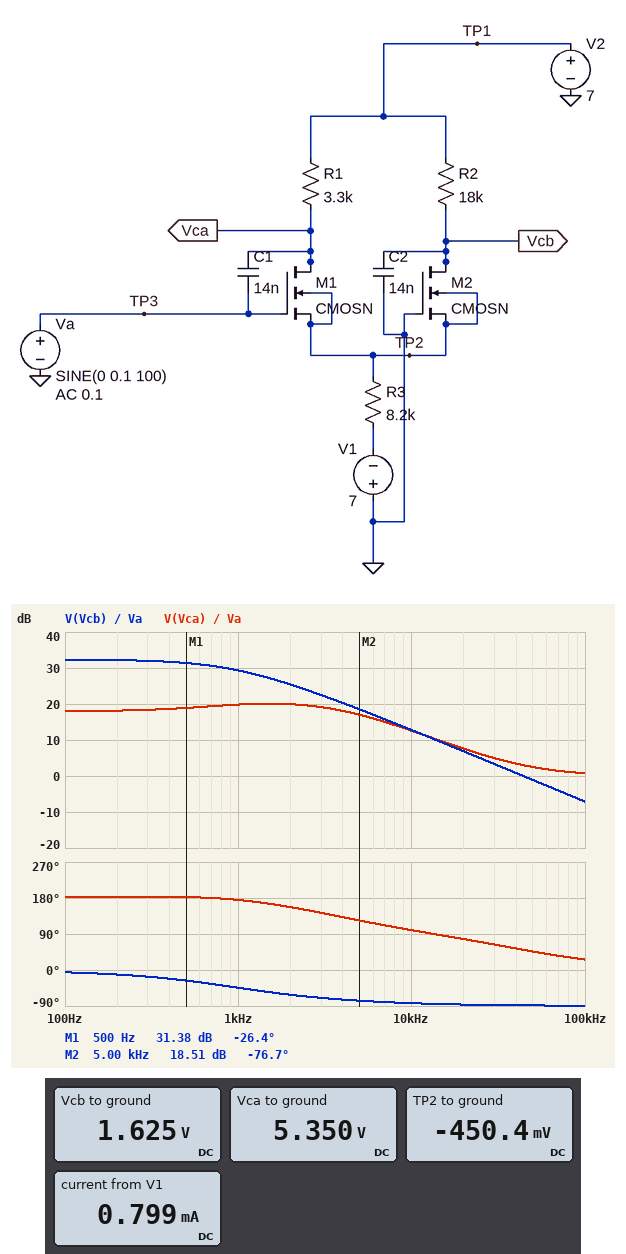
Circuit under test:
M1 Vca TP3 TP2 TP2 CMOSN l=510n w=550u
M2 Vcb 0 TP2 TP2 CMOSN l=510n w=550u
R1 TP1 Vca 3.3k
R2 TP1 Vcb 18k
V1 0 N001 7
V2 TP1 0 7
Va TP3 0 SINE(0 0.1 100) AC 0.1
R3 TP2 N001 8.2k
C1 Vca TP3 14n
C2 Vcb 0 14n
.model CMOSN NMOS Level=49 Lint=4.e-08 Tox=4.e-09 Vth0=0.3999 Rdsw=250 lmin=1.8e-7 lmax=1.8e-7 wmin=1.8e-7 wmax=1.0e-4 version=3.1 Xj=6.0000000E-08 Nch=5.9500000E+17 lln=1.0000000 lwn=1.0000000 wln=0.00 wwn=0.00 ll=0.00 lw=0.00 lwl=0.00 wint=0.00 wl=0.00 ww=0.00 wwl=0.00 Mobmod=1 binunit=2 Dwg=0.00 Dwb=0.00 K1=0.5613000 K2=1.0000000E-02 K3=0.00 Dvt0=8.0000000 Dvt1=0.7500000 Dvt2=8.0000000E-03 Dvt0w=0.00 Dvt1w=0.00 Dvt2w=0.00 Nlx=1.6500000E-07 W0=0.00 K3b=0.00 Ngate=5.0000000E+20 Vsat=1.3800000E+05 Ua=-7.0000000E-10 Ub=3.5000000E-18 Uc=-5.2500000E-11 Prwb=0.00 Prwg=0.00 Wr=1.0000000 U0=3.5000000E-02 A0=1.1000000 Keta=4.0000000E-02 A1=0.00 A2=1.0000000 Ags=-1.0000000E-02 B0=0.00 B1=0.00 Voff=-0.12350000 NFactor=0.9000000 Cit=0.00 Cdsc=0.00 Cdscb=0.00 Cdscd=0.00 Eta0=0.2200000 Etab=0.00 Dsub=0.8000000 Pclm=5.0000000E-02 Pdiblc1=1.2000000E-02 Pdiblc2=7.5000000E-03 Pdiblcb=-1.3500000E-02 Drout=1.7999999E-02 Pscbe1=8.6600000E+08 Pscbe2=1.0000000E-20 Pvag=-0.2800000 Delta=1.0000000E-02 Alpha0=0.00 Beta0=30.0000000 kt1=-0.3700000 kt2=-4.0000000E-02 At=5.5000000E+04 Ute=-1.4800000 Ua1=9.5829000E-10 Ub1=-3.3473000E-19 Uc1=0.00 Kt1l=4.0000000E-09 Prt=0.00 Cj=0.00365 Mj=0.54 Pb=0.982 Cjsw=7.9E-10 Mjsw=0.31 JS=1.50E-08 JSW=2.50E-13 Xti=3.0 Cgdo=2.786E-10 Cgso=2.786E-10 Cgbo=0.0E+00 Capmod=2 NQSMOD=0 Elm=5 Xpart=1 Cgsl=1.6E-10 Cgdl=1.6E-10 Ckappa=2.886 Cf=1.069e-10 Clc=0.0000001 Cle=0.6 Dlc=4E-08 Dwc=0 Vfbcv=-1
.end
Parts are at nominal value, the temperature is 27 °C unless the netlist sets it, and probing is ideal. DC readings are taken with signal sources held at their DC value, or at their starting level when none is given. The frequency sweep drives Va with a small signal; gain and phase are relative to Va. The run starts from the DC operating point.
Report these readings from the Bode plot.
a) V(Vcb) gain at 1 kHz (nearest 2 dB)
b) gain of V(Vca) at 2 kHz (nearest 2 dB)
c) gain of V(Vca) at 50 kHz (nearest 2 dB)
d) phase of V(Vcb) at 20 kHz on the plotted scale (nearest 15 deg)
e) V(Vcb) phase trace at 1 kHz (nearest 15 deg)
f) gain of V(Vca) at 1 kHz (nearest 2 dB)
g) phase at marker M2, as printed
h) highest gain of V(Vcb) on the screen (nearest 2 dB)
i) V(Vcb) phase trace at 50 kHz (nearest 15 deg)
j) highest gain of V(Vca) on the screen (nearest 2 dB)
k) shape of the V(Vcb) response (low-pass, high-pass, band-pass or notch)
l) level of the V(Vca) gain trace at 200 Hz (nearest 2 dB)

30 dB
20 dB
2 dB
-90 deg
-45 deg
20 dB
-76.7 deg
32 dB
-90 deg
20 dB
low-pass
18 dB
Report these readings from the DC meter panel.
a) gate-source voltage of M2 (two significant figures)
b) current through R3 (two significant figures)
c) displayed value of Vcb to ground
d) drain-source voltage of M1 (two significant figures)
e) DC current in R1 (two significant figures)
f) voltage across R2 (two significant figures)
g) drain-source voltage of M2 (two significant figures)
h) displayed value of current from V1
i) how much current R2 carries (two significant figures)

450 mV
800 µA
1.625 V
5.8 V
500 µA
5.4 V
2.1 V
0.799 mA
300 µA
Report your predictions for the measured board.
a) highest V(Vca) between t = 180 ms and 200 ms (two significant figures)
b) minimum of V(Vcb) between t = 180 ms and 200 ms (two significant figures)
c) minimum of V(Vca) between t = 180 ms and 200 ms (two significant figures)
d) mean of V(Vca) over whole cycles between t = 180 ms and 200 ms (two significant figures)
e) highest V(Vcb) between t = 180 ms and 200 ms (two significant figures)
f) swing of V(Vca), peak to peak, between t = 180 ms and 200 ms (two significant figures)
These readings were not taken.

5.8 V
-510 mV
4.6 V
5.3 V
5.4 V
1.2 V
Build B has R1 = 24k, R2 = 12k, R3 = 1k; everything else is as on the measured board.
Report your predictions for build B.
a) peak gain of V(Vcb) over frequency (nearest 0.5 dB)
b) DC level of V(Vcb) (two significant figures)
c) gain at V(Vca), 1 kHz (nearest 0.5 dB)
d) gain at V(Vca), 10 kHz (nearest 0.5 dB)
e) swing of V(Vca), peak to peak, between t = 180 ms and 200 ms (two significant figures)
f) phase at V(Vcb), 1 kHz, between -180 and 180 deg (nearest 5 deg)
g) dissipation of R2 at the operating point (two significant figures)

-6.0 dB
-5.4 V
-22.0 dB
-7.5 dB
1.6 mV
80 deg
13 mW
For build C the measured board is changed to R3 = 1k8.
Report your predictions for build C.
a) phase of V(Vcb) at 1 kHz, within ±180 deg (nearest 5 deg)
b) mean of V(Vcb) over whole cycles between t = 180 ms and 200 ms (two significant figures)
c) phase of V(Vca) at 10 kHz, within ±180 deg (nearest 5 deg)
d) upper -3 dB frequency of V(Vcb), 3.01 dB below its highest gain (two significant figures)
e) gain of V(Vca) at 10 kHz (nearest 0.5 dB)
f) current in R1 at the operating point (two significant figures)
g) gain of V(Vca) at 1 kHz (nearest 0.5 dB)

80 deg
-1.5 V
30 deg
2.6 MHz
-7.0 dB
2.6 mA
-20.5 dB
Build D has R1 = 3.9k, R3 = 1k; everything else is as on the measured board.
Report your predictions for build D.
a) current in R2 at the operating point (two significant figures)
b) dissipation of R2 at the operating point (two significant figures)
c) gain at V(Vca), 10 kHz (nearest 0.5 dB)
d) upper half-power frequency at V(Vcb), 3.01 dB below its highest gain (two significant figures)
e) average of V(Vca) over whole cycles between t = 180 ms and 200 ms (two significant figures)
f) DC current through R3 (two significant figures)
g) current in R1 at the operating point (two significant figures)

590 µA
6.3 mW
-8.0 dB
3.0 MHz
-3.7 V
3.3 mA
2.7 mA
